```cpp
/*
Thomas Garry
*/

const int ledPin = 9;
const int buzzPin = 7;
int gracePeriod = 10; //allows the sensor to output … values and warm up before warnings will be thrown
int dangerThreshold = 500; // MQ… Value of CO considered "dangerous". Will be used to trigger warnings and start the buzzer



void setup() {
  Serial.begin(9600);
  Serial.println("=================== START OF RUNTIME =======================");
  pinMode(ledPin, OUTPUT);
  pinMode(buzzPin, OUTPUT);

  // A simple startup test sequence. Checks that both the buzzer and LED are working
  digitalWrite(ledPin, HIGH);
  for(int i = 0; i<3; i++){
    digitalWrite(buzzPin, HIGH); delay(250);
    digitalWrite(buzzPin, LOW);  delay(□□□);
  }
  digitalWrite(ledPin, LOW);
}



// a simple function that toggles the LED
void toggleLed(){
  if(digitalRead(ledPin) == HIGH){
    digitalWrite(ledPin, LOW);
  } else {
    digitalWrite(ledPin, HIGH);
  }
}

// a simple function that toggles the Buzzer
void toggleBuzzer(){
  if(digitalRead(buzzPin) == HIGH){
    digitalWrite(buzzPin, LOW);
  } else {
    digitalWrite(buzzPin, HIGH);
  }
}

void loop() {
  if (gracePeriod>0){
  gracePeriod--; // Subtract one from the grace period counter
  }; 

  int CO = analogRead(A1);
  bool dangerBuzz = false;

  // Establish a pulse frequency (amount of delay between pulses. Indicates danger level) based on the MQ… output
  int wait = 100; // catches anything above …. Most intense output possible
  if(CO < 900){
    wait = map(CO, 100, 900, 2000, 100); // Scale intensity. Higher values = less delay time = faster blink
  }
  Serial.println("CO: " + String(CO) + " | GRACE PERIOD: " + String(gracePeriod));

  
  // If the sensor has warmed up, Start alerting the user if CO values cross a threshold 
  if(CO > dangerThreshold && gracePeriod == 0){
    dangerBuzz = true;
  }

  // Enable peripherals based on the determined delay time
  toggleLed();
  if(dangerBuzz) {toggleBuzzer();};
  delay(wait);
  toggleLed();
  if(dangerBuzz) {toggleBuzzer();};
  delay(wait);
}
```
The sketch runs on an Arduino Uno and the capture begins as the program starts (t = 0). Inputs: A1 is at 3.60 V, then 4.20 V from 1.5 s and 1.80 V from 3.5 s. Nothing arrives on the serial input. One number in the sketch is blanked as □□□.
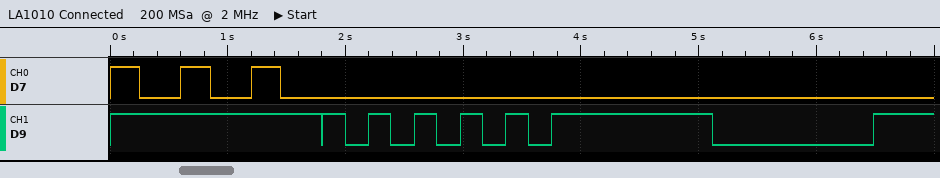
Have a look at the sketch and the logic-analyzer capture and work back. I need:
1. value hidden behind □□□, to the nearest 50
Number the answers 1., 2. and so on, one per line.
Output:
1. 350
